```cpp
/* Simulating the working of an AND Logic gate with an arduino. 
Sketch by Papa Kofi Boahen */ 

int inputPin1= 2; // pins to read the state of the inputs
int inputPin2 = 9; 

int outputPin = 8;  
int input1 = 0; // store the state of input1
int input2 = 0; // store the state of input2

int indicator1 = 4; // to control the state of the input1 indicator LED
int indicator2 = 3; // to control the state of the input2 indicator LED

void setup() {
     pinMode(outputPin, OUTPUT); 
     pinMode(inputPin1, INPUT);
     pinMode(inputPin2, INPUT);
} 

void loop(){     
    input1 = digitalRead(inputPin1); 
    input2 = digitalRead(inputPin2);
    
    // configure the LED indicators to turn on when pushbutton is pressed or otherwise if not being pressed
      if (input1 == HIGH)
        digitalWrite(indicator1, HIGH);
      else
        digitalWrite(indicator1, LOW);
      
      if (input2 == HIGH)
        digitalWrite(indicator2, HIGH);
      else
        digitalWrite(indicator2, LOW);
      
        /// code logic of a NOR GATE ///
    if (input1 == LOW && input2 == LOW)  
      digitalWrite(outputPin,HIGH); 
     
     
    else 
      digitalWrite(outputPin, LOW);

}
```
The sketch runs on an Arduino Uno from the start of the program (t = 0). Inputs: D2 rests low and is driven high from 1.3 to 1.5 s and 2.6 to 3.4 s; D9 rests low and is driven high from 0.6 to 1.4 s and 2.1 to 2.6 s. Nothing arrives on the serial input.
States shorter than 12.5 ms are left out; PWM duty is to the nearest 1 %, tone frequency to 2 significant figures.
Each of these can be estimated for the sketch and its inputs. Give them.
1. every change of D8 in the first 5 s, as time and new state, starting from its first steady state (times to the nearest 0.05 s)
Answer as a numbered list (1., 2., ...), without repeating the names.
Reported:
1. 0 s high; 0.6 s low; 1.5 s high; 2.1 s low; 3.4 s high
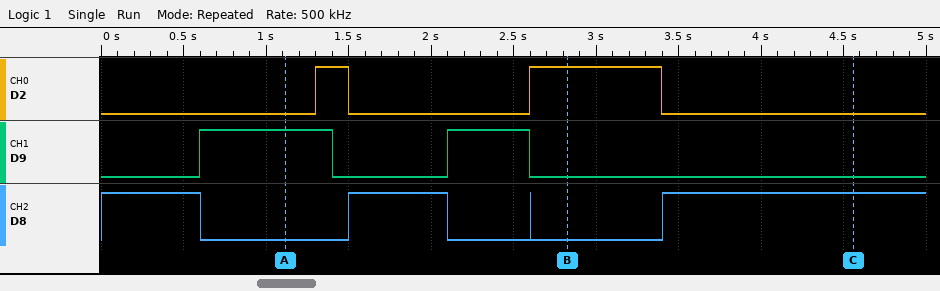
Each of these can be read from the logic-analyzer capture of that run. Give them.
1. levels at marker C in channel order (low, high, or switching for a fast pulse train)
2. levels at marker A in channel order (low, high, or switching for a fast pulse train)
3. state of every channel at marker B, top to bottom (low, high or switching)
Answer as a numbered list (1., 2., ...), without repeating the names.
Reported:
1. D2 low, D9 low, D8 high
2. D2 low, D9 high, D8 low
3. D2 high, D9 low, D8 low
